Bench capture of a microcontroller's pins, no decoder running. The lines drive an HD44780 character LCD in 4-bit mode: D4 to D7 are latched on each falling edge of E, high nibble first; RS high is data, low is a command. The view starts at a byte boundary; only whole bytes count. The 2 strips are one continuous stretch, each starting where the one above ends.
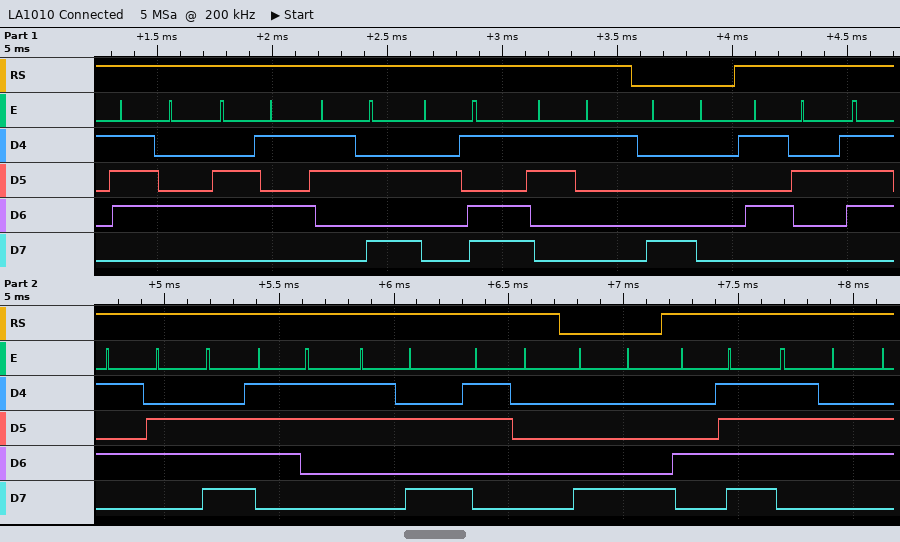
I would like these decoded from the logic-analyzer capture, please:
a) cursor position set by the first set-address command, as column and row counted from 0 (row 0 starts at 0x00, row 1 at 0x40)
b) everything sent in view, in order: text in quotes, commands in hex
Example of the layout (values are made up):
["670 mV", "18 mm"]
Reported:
["column 0, row 0", "\"te:-1\" 0x80 \"Runs:0\" 0x88 \"Ov\""]
